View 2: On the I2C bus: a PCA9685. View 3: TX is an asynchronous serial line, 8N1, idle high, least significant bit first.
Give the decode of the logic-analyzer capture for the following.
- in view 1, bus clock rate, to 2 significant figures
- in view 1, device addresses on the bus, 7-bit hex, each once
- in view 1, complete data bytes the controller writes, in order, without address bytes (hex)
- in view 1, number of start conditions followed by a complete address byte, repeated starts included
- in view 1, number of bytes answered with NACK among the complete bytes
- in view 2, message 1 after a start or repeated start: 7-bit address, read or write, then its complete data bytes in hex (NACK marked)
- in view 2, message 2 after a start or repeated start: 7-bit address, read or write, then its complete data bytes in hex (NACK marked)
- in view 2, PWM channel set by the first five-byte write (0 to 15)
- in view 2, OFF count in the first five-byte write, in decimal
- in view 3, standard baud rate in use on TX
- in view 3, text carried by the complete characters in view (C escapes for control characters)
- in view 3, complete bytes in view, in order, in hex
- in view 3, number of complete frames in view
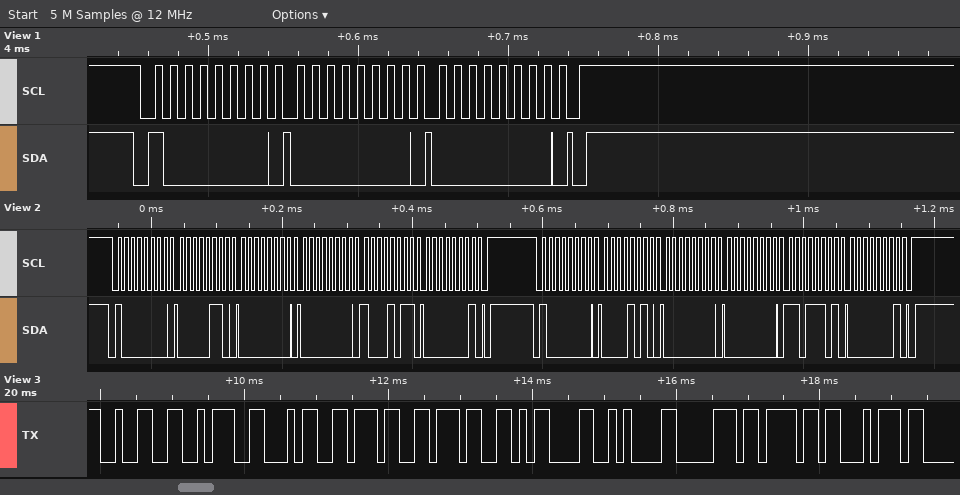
100 kHz
0x40
00 00
1
0
0x40 write: 06 00 00 8B 01
0x40 write: 0A 00 00 DD 01
0
395
9600 baud
"2:477\r\npot"
32 3A 34 37 37 0D 0A 70 6F 74
10
